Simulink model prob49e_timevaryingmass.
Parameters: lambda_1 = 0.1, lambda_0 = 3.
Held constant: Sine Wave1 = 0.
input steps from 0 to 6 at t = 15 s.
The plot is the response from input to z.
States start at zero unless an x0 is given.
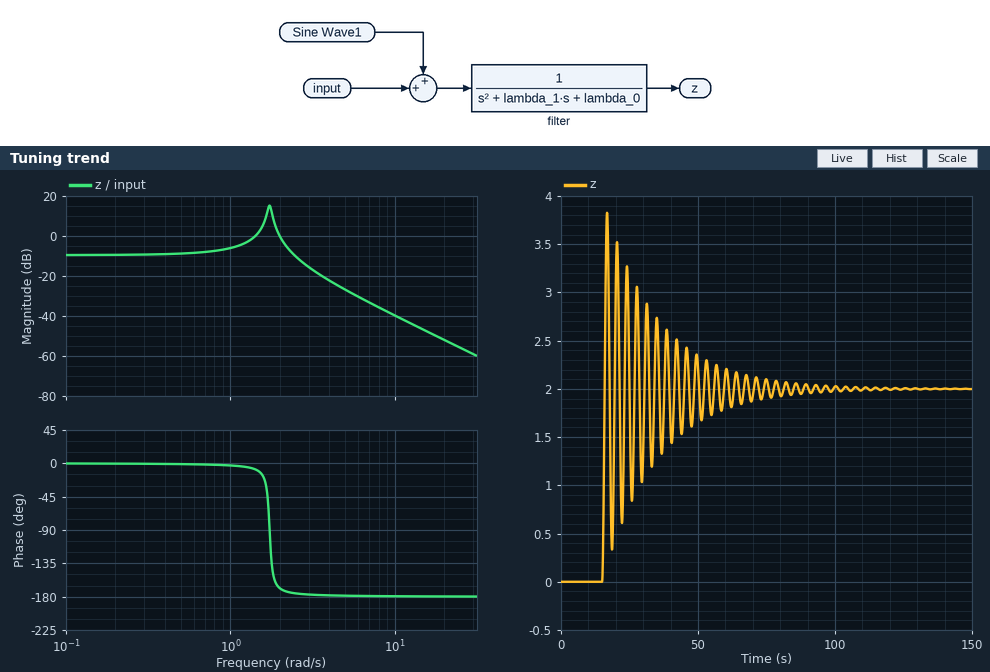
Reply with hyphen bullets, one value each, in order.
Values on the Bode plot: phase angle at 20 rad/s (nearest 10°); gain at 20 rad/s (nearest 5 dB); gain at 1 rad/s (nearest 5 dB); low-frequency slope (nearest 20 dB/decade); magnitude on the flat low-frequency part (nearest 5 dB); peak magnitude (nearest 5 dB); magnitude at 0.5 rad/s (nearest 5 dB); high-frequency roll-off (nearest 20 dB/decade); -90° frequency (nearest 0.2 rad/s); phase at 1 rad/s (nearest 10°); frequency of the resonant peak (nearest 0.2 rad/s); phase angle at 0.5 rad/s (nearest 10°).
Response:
- -180°
- -50 dB
- -5 dB
- 0 dB/decade
- -10 dB
- 15 dB
- -10 dB
- -40 dB/decade
- 1.8 rad/s
- 0°
- 1.8 rad/s
- 0°
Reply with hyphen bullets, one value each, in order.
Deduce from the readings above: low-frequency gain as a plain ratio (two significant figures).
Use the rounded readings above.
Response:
- 0.32
